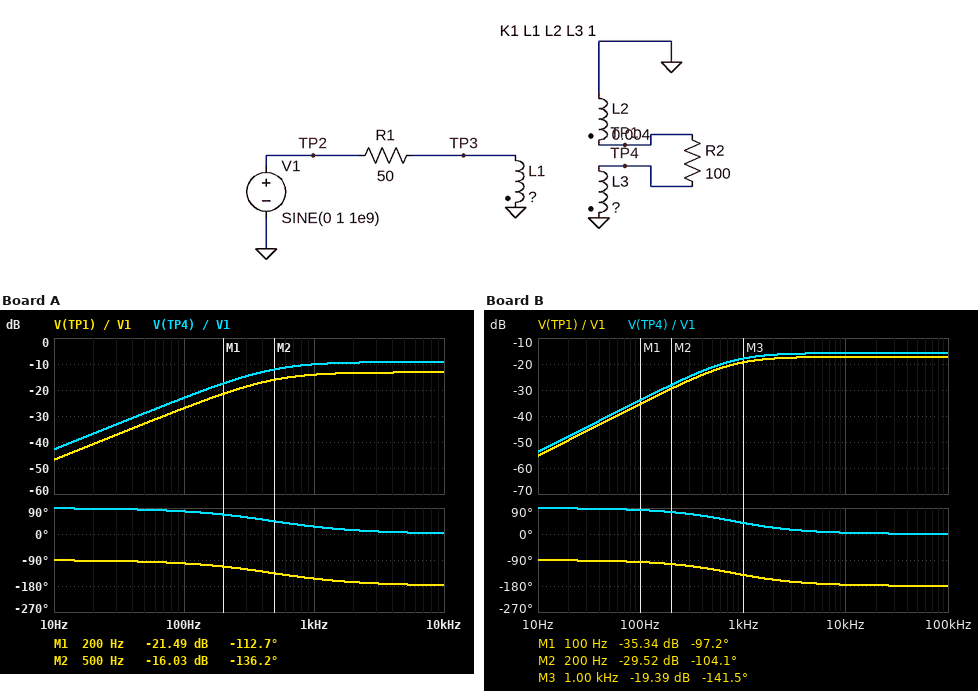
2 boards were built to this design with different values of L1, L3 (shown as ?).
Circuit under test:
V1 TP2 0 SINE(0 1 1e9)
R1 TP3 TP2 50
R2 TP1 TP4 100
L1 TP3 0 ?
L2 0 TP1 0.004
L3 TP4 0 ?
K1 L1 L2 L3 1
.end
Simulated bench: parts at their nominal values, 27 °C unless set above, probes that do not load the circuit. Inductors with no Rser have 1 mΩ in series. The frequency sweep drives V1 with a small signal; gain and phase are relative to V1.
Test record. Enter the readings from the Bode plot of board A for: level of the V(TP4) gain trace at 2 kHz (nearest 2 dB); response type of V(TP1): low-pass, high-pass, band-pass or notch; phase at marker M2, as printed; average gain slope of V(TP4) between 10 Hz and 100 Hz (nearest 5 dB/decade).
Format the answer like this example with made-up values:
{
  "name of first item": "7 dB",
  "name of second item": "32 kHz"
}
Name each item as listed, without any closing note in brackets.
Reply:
{
  "level of the V(TP4) gain trace at 2 kHz": "-10 dB",
  "response type of V(TP1): low-pass, high-pass, band-pass or notch": "high-pass",
  "phase at marker M2, as printed": "-136.2 deg",
  "average gain slope of V(TP4) between 10 Hz and 100 Hz": "20 dB/decade"
}
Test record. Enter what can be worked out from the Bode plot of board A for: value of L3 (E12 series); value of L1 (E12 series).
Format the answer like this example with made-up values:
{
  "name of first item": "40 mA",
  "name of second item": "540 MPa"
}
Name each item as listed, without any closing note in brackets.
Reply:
{
  "value of L3": "10 mH",
  "value of L1": "3.3 mH"
}
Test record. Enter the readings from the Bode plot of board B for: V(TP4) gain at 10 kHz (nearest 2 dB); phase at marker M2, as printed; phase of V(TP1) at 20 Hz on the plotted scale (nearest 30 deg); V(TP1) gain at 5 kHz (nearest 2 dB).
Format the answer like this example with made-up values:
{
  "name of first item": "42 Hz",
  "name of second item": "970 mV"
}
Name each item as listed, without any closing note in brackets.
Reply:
{
  "V(TP4) gain at 10 kHz": "-16 dB",
  "phase at marker M2, as printed": "-104.1 deg",
  "phase of V(TP1) at 20 Hz on the plotted scale": "-90 deg",
  "V(TP1) gain at 5 kHz": "-18 dB"
}
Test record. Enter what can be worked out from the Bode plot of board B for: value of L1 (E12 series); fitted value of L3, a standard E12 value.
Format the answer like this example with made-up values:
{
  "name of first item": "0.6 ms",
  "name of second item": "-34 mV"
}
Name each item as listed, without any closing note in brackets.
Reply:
{
  "value of L1": "470 µH",
  "fitted value of L3, a standard E12 value": "5.6 mH"
}
